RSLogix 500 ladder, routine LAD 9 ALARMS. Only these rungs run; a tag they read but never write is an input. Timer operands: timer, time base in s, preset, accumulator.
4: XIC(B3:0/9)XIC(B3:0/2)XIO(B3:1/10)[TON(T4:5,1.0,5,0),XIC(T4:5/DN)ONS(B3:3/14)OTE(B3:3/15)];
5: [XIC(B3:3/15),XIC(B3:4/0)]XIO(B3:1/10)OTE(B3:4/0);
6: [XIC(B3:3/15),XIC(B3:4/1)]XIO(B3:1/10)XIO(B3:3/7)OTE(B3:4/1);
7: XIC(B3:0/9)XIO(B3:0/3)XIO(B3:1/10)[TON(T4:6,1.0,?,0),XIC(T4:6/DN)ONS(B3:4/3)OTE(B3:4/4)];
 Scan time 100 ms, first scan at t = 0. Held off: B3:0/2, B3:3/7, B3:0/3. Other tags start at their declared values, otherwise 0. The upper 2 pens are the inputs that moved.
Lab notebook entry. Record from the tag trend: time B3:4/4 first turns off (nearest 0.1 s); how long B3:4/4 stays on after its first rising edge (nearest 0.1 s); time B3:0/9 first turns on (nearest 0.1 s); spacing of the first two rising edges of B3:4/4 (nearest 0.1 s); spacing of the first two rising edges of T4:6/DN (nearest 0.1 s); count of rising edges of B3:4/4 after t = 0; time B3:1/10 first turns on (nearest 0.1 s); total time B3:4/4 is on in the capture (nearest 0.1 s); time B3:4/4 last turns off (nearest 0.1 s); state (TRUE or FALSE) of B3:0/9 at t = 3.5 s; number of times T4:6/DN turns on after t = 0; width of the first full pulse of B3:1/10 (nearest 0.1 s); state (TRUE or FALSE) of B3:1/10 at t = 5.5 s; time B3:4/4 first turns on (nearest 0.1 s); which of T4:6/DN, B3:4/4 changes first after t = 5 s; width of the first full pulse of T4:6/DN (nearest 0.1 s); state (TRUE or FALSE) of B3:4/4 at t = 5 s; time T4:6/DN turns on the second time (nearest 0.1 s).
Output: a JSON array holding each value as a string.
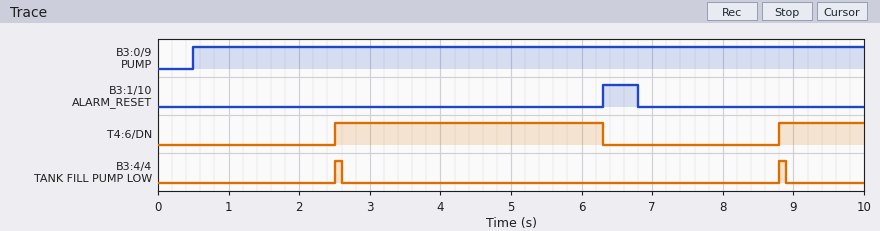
["2.6 s", "0.1 s", "0.5 s", "6.3 s", "6.3 s", "2", "6.3 s", "0.2 s", "8.9 s", "TRUE", "2", "0.5 s", "FALSE", "2.5 s", "T4:6/DN", "3.8 s", "FALSE", "8.8 s"]
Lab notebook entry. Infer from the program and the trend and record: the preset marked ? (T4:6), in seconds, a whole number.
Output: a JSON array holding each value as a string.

["2 s"]
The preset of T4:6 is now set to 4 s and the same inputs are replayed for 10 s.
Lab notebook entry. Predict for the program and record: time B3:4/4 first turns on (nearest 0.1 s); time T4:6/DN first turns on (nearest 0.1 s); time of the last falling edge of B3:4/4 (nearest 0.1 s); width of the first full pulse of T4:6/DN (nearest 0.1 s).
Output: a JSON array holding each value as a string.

["4.5 s", "4.5 s", "4.6 s", "1.8 s"]
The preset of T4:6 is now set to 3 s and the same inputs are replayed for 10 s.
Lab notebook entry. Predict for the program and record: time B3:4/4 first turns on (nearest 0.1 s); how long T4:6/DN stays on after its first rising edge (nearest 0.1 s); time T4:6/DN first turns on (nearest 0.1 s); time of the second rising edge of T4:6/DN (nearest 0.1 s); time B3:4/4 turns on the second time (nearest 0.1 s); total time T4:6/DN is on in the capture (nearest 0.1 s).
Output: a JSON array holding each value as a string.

["3.5 s", "2.8 s", "3.5 s", "9.8 s", "9.8 s", "3.0 s"]
